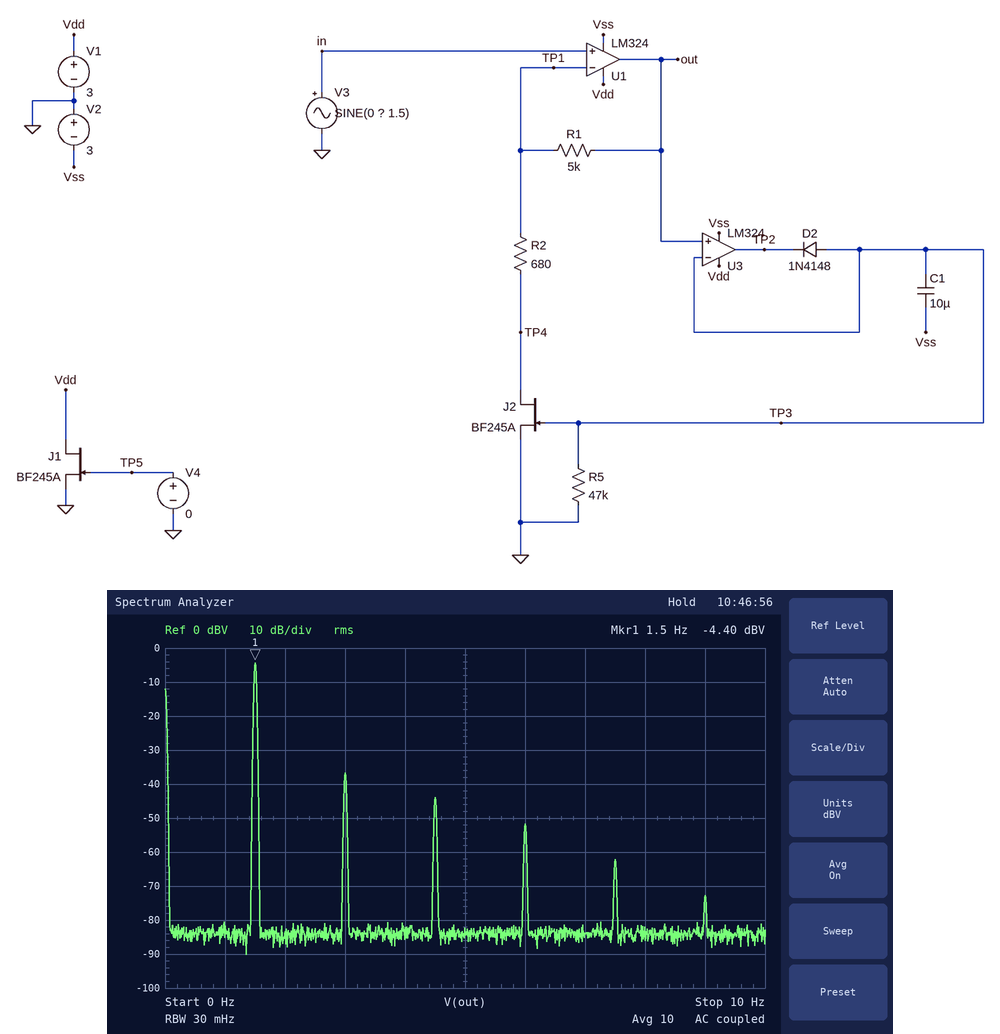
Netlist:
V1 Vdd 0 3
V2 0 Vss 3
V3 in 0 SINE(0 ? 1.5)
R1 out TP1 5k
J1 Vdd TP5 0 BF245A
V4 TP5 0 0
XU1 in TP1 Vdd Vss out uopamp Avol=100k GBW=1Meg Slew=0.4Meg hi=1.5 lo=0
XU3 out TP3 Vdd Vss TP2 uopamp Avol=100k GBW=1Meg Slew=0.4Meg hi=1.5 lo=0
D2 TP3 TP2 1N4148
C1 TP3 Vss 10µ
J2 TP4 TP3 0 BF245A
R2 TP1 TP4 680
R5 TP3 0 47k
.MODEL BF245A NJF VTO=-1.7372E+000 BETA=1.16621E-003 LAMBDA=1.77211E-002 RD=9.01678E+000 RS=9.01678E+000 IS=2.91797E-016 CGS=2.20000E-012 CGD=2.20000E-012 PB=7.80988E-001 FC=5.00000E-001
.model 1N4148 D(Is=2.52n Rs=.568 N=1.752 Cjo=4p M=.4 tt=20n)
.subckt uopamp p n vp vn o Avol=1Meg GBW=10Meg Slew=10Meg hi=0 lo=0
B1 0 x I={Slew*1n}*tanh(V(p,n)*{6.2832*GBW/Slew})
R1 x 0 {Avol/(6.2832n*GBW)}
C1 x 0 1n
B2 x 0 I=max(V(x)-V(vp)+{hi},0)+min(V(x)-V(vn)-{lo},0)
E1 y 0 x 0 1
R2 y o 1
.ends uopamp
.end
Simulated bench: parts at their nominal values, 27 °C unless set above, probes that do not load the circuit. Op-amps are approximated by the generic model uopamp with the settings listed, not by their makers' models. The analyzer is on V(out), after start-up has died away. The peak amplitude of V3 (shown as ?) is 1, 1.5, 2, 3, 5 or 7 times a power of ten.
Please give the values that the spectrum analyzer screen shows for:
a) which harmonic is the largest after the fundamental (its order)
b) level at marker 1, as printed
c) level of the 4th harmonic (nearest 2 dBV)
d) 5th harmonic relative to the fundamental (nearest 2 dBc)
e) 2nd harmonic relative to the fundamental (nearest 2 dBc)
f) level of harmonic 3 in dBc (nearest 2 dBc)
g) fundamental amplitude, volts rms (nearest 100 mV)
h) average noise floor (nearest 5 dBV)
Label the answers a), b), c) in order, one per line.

a) 2
b) -4.40 dBV
c) -52 dBV
d) -58 dBc
e) -32 dBc
f) -40 dBc
g) 600 mV
h) -85 dBV
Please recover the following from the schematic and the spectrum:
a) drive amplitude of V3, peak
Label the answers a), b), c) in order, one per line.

a) 150 mV
